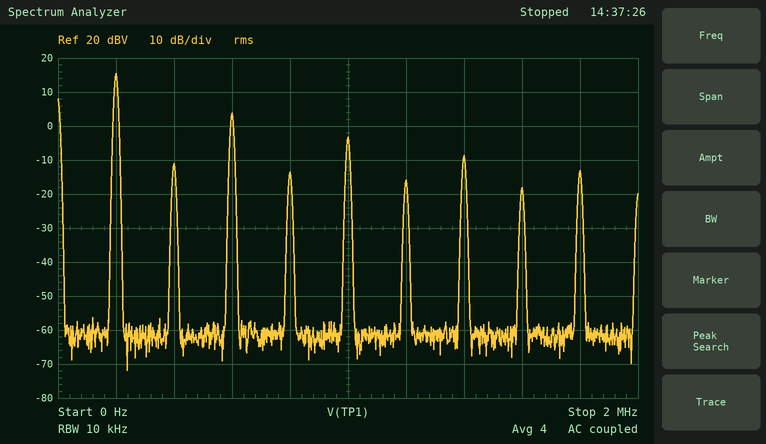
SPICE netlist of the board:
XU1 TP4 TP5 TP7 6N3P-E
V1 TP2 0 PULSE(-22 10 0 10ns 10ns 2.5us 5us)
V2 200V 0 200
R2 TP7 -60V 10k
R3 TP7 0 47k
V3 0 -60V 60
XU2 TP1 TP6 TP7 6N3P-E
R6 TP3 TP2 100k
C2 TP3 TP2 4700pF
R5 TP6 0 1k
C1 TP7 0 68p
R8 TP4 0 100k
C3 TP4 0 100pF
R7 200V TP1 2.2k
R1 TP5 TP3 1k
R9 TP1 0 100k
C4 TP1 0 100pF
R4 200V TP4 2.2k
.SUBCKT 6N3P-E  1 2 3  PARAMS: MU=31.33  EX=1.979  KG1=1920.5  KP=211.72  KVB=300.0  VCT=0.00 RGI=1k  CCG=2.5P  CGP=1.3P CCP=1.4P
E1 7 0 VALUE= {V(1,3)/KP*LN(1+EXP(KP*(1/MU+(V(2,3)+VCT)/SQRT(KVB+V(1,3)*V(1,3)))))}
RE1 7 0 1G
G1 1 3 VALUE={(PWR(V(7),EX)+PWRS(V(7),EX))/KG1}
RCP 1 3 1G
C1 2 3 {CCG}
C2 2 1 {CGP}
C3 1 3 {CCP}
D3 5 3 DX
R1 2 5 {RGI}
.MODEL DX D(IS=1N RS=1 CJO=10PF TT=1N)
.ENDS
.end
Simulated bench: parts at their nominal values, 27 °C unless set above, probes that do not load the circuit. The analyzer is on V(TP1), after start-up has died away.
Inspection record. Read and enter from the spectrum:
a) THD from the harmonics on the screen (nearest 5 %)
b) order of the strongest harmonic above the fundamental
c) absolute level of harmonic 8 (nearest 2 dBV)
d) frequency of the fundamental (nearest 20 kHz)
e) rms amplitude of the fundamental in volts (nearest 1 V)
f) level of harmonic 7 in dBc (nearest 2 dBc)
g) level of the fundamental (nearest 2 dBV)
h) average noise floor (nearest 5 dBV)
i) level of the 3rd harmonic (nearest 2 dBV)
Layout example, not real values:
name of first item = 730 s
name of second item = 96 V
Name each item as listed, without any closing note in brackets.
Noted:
THD from the harmonics on the screen = 30 %
order of the strongest harmonic above the fundamental = 3
absolute level of harmonic 8 = -18 dBV
frequency of the fundamental = 200 kHz
rms amplitude of the fundamental in volts = 6 V
level of harmonic 7 in dBc = -24 dBc
level of the fundamental = 16 dBV
average noise floor = -60 dBV
level of the 3rd harmonic = 4 dBV
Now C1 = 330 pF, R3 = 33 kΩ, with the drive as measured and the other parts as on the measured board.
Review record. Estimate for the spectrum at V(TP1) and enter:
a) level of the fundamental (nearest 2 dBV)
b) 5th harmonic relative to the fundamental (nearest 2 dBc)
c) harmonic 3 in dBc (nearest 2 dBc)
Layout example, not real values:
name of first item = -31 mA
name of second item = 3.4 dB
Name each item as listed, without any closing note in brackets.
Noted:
level of the fundamental = 16 dBV
5th harmonic relative to the fundamental = -28 dBc
harmonic 3 in dBc = -14 dBc
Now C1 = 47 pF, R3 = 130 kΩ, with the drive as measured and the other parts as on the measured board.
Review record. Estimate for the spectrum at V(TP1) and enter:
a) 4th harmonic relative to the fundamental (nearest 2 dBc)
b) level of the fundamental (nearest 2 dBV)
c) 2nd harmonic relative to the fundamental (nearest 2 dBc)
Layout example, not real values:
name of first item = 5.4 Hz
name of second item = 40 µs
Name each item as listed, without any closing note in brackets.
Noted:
4th harmonic relative to the fundamental = -32 dBc
level of the fundamental = 16 dBV
2nd harmonic relative to the fundamental = -30 dBc
